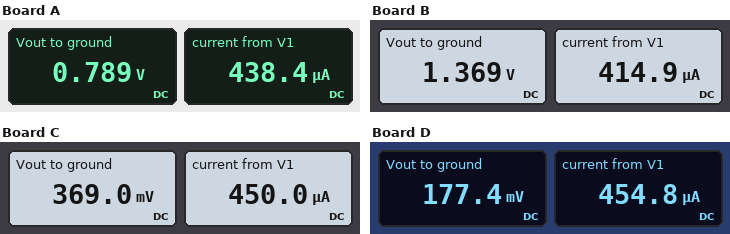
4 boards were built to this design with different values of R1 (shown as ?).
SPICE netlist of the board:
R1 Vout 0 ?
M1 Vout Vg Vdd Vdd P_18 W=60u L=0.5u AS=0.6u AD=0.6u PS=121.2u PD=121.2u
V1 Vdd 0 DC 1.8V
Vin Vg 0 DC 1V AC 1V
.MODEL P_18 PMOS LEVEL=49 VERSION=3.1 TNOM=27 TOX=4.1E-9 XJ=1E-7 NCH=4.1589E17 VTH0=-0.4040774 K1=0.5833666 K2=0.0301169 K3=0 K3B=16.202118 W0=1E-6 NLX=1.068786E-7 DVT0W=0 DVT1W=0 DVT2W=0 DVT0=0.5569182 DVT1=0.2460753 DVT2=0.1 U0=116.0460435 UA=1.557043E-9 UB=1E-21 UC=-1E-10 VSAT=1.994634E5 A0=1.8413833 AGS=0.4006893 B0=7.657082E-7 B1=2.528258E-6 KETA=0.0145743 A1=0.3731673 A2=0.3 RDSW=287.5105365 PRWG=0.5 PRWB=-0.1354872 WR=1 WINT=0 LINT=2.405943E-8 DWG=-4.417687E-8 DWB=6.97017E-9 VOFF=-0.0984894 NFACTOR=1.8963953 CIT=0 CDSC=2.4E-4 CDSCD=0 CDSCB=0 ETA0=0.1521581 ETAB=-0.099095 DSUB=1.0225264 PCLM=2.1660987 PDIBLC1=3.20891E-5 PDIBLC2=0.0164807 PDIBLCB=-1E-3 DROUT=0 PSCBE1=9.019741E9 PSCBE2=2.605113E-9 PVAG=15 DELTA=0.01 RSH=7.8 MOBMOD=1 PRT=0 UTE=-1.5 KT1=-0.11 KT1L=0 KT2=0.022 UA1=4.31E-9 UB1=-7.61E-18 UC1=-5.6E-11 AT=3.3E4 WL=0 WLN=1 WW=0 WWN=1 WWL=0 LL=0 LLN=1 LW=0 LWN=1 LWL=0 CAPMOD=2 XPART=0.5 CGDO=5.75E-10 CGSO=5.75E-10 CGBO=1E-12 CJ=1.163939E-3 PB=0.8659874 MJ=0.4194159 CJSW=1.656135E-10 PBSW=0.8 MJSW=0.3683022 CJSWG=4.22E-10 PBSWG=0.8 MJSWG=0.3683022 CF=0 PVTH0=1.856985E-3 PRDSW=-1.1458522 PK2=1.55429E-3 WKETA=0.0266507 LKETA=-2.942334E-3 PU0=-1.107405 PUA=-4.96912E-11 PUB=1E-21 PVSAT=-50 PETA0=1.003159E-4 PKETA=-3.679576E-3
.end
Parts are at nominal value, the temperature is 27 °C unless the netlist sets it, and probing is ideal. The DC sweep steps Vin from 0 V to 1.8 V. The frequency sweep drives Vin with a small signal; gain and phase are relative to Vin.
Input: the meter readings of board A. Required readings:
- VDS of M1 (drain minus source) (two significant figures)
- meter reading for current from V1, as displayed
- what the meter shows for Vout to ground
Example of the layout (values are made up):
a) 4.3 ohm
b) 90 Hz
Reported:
a) -1.0 V
b) 438.4 µA
c) 0.789 V
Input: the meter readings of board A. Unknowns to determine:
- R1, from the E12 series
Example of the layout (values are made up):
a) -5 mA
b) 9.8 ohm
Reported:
a) 1.8 kΩ
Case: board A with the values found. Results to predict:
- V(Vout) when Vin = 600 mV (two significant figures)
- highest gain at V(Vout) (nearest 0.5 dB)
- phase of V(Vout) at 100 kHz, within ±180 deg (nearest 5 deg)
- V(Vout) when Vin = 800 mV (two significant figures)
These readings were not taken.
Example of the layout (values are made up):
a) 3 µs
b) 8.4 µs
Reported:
a) 1.6 V
b) 11.5 dB
c) 150 deg
d) 1.5 V
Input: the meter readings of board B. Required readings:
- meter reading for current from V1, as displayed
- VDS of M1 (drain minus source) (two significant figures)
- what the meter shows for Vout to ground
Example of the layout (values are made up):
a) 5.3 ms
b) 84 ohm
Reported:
a) 414.9 µA
b) -430 mV
c) 1.369 V
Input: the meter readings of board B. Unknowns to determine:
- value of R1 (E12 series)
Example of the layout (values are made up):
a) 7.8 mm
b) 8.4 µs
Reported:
a) 3.3 kΩ
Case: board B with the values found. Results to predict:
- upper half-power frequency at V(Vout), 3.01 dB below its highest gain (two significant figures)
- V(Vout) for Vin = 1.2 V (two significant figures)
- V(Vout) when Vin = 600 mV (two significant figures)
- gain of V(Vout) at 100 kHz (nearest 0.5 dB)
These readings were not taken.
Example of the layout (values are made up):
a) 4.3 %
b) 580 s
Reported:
a) 99 kHz
b) 320 mV
c) 1.7 V
d) 12.0 dB
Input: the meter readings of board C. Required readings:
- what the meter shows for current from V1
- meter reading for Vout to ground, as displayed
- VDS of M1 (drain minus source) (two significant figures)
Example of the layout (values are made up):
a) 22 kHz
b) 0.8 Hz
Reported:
a) 450.0 µA
b) 369.0 mV
c) -1.4 V
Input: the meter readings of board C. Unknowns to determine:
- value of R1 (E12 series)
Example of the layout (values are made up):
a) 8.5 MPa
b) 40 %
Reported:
a) 820 Ω
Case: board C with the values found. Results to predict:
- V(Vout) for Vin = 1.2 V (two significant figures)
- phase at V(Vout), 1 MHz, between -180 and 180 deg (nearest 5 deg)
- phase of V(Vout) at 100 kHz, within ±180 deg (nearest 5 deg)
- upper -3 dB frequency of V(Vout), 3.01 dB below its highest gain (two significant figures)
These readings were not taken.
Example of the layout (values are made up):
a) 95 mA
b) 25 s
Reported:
a) 82 mV
b) 115 deg
c) 165 deg
d) 420 kHz
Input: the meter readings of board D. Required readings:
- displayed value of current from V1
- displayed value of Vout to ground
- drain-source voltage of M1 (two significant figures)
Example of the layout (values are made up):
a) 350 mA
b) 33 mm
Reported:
a) 454.8 µA
b) 177.4 mV
c) -1.6 V
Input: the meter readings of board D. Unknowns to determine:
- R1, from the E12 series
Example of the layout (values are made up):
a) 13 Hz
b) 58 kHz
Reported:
a) 390 Ω
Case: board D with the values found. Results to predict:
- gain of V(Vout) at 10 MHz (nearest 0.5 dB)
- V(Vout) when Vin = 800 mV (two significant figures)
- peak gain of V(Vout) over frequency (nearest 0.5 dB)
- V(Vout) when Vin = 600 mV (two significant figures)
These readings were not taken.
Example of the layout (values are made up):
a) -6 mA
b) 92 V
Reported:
a) -22.0 dB
b) 390 mV
c) -1.0 dB
d) 650 mV
